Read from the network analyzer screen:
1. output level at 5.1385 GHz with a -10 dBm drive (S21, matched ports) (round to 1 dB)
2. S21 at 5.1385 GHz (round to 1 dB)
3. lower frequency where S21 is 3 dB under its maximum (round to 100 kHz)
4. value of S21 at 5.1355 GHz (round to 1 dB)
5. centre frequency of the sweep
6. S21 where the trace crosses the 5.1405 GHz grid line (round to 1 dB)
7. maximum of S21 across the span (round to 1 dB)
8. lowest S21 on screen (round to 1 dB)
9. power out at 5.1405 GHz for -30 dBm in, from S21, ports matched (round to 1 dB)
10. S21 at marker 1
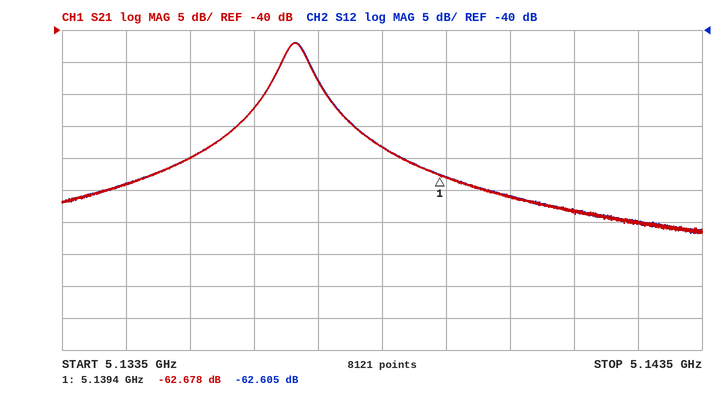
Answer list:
-68 dBm
-58 dB
5.1369 GHz
-60 dB
5.1385 GHz
-66 dB
-42 dB
-72 dB
-96 dBm
-62.678 dB
